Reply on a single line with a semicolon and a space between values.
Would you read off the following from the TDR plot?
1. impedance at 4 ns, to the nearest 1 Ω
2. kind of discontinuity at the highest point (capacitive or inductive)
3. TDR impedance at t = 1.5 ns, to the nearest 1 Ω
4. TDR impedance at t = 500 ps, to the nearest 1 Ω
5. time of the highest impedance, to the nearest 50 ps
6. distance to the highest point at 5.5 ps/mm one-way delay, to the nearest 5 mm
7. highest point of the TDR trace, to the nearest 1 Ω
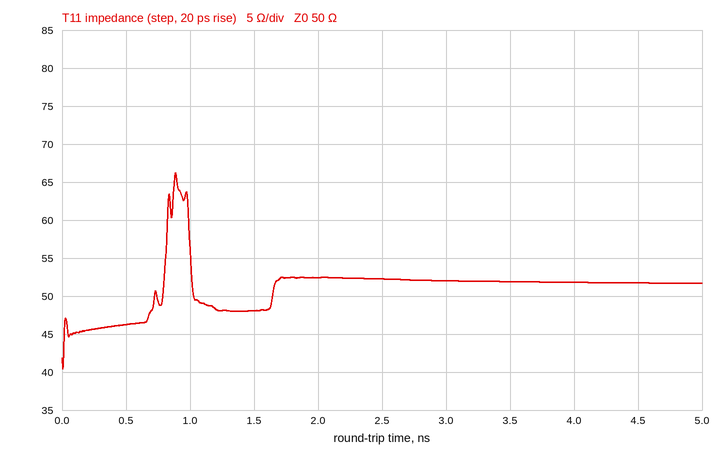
52 Ω; inductive; 48 Ω; 46 Ω; 900 ps; 80 mm; 66 Ω
